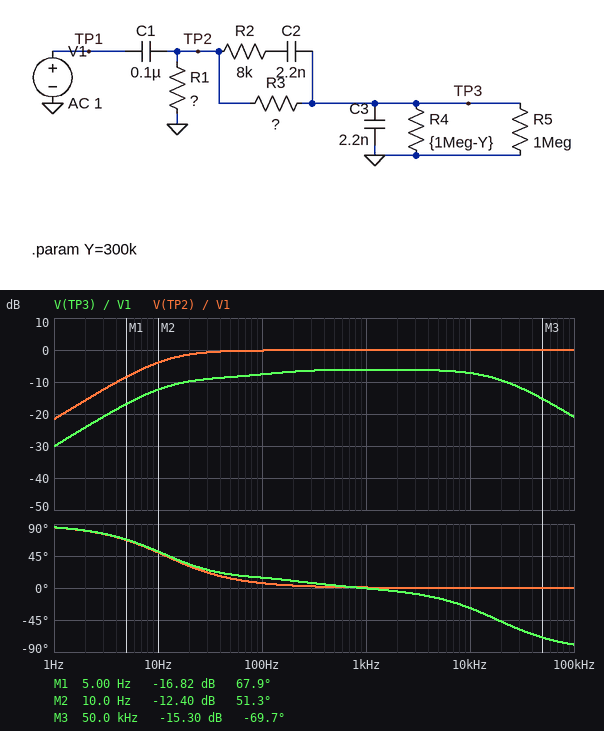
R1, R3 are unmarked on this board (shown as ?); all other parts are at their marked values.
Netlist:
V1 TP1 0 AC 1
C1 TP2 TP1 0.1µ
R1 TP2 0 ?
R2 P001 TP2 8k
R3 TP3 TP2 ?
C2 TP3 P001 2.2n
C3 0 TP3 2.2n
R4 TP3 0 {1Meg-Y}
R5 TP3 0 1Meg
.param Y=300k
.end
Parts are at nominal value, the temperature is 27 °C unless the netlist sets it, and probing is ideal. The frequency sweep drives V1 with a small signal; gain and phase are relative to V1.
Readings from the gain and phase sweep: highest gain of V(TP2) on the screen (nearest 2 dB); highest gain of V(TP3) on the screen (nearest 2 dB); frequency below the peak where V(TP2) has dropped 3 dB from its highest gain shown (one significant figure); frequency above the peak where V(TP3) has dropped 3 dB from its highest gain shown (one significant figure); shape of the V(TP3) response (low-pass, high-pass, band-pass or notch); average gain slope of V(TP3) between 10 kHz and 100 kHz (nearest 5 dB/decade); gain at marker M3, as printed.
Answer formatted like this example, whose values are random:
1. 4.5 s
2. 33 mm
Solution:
1. 0 dB
2. -6 dB
3. 10 Hz
4. 20 kHz
5. band-pass
6. -15 dB/decade
7. -15.30 dB
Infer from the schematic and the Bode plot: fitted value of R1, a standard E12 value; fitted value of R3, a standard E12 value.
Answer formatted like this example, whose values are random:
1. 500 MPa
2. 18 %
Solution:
1. 150 kΩ
2. 680 kΩ
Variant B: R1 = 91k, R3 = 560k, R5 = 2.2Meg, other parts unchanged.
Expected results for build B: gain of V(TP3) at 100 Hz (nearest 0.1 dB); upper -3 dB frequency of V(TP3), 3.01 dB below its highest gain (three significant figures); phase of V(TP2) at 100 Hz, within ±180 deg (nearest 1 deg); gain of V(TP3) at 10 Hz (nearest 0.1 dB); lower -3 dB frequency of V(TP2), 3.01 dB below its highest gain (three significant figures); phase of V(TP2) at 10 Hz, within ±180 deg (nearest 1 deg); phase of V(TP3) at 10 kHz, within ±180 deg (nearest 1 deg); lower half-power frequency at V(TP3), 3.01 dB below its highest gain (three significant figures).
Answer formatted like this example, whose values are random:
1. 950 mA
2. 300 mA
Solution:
1. -6.4 dB
2. 18.5 kHz
3. 11 deg
4. -12.9 dB
5. 19.2 Hz
6. 62 deg
7. -28 deg
8. 20.0 Hz
